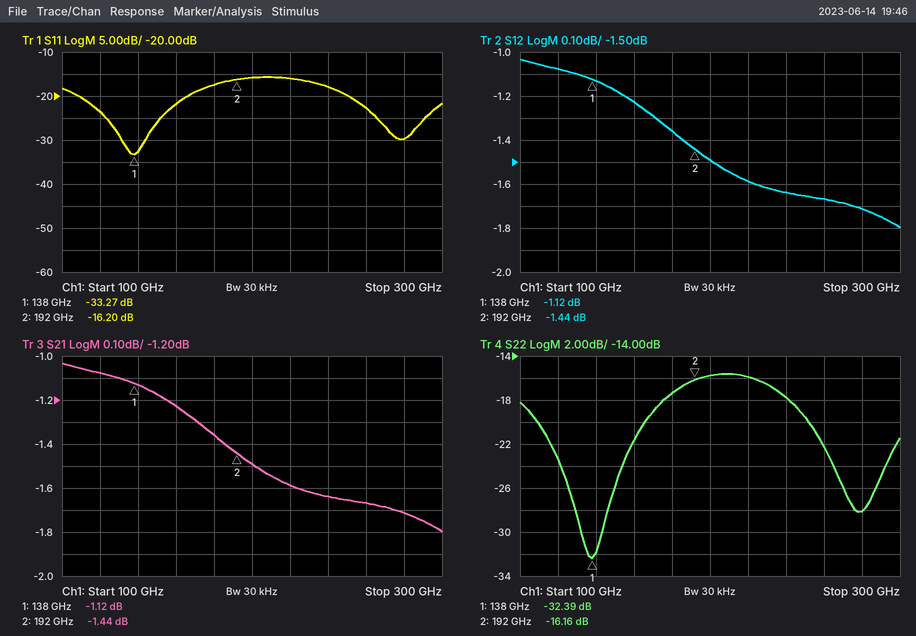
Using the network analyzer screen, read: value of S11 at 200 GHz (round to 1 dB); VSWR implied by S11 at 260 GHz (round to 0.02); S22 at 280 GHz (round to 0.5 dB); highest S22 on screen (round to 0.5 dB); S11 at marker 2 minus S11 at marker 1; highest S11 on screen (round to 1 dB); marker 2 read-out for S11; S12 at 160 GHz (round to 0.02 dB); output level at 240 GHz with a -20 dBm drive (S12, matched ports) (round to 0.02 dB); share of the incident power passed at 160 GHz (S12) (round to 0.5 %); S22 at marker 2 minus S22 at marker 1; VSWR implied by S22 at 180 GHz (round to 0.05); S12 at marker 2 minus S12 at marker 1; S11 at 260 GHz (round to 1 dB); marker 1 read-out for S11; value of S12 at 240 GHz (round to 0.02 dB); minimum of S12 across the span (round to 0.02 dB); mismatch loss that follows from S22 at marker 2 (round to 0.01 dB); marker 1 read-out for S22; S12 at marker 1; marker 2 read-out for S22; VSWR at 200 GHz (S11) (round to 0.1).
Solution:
-16 dB
1.16
-28.0 dB
-15.5 dB
17.07 dB
-16 dB
-16.20 dB
-1.22 dB
-21.64 dBm
75.5 %
16.23 dB
1.30
-0.32 dB
-23 dB
-33.27 dB
-1.64 dB
-1.80 dB
0.11 dB
-32.39 dB
-1.12 dB
-16.16 dB
1.4
